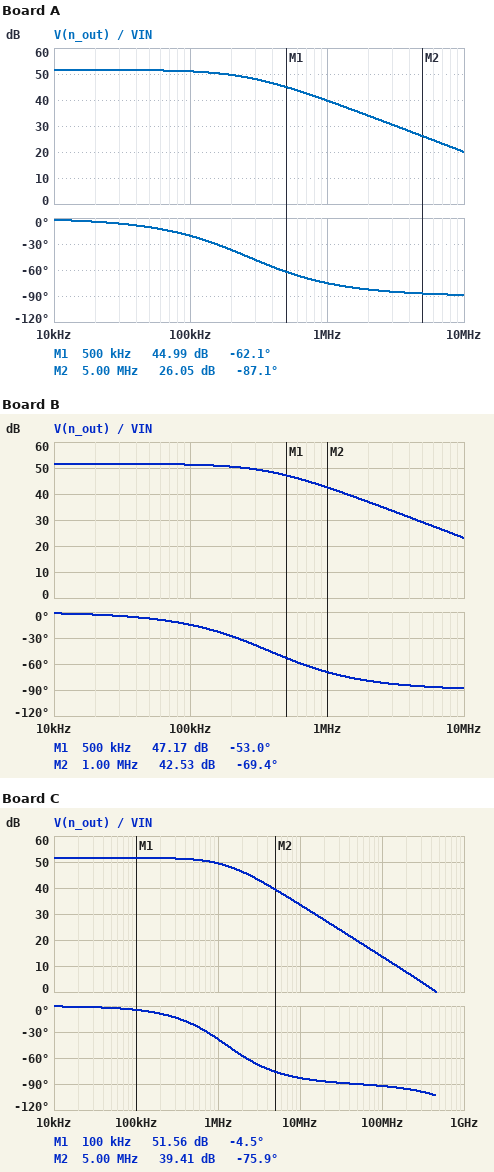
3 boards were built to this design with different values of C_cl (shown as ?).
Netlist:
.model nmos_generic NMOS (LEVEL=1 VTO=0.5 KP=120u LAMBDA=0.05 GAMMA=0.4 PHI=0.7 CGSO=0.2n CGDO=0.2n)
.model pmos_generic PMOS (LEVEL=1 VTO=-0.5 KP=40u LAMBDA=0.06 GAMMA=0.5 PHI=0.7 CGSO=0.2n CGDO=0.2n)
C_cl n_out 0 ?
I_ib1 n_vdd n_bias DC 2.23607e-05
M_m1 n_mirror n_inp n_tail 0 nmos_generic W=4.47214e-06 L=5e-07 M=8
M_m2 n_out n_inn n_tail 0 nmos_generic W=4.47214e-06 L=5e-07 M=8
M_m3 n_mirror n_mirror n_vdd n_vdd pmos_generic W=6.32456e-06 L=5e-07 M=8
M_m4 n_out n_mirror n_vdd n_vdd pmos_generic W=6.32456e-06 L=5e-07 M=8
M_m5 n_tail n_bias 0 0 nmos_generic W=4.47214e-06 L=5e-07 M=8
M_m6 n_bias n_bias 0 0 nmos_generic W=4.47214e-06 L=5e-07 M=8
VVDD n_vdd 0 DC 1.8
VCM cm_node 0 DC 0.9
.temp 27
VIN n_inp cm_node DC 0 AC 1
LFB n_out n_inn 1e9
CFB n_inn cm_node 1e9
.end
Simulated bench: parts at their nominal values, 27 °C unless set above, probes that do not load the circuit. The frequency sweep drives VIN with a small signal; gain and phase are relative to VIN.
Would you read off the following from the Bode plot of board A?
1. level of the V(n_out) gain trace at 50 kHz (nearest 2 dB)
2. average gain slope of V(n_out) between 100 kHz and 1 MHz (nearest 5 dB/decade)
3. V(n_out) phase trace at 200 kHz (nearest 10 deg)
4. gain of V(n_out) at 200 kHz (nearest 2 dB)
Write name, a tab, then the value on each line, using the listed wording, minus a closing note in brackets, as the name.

level of the V(n_out) gain trace at 50 kHz	52 dB
average gain slope of V(n_out) between 100 kHz and 1 MHz	-10 dB/decade
V(n_out) phase trace at 200 kHz	-40 deg
gain of V(n_out) at 200 kHz	50 dB
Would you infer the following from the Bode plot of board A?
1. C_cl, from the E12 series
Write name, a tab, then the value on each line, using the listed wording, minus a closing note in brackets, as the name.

C_cl, from the E12 series	680 fF
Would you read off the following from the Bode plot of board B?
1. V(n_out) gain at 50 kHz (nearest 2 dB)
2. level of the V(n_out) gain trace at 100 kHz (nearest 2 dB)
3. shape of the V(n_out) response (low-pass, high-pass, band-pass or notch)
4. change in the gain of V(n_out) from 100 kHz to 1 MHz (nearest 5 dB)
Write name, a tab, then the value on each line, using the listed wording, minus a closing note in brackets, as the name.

V(n_out) gain at 50 kHz	52 dB
level of the V(n_out) gain trace at 100 kHz	52 dB
shape of the V(n_out) response	low-pass
change in the gain of V(n_out) from 100 kHz to 1 MHz	-10 dB
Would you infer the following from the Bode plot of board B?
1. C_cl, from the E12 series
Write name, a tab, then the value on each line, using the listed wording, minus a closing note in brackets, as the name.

C_cl, from the E12 series	470 fF
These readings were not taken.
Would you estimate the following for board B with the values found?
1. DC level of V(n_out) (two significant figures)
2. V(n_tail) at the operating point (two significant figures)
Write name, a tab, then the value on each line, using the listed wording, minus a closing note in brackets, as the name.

DC level of V(n_out)	900 mV
V(n_tail) at the operating point	290 mV
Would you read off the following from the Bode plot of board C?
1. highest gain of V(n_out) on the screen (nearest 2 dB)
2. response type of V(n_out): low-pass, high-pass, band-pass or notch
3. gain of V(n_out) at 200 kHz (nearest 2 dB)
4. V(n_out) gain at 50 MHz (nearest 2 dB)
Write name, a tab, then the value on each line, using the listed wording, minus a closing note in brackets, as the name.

highest gain of V(n_out) on the screen	52 dB
response type of V(n_out): low-pass, high-pass, band-pass or notch	low-pass
gain of V(n_out) at 200 kHz	52 dB
V(n_out) gain at 50 MHz	20 dB
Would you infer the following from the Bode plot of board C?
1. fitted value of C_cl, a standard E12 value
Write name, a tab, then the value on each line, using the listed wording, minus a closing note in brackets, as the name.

fitted value of C_cl, a standard E12 value	120 fF
